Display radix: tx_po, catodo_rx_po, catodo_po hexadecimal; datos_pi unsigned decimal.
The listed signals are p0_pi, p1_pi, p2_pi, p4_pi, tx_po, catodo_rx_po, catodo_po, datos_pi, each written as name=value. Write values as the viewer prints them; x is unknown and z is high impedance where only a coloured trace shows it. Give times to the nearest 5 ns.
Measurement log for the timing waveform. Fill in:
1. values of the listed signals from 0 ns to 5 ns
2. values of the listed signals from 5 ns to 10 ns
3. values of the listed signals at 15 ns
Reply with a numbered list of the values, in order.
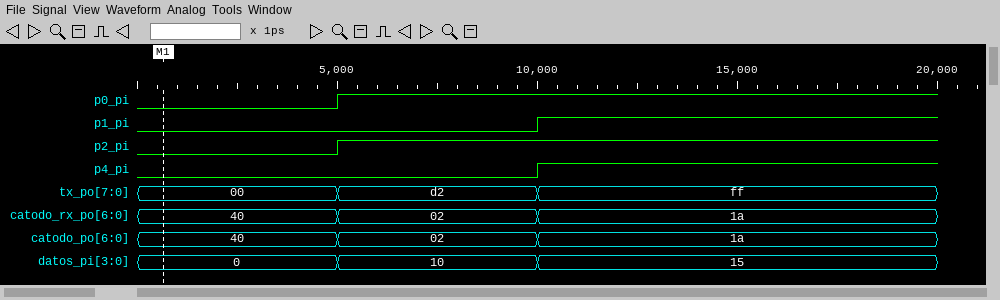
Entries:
1. p0_pi=0, p1_pi=0, p2_pi=0, p4_pi=0, tx_po=00, catodo_rx_po=40, catodo_po=40, datos_pi=0
2. p0_pi=1, p1_pi=0, p2_pi=1, p4_pi=0, tx_po=d2, catodo_rx_po=02, catodo_po=02, datos_pi=10
3. p0_pi=1, p1_pi=1, p2_pi=1, p4_pi=1, tx_po=ff, catodo_rx_po=1a, catodo_po=1a, datos_pi=15
